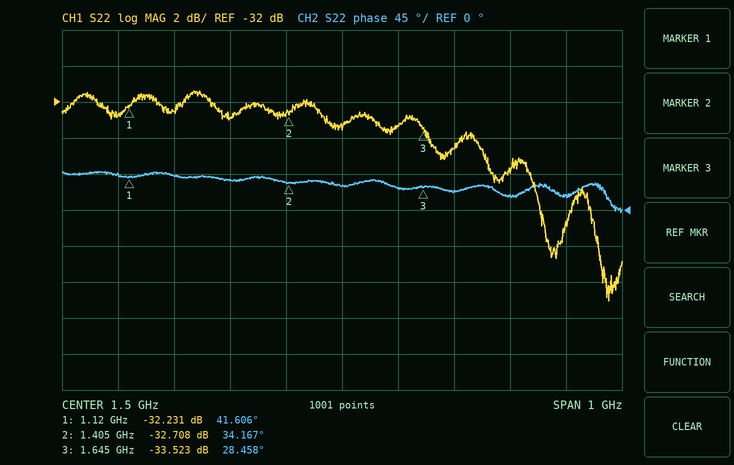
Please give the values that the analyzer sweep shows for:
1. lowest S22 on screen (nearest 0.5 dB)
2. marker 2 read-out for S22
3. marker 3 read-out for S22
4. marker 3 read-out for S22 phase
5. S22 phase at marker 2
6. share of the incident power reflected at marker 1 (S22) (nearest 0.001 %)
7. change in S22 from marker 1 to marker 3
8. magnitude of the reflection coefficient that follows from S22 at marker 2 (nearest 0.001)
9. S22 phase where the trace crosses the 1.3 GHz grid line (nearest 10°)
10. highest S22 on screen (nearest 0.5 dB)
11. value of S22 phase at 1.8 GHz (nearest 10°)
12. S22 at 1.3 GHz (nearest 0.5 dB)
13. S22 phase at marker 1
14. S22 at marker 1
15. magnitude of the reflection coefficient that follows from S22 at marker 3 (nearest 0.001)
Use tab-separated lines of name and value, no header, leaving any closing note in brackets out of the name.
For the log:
lowest S22 on screen	-43.0 dB
marker 2 read-out for S22	-32.708 dB
marker 3 read-out for S22	-33.523 dB
marker 3 read-out for S22 phase	28.458°
S22 phase at marker 2	34.167°
share of the incident power reflected at marker 1 (S22)	0.060 %
change in S22 from marker 1 to marker 3	-1.292 dB
magnitude of the reflection coefficient that follows from S22 at marker 2	0.023
S22 phase where the trace crosses the 1.3 GHz grid line	40°
highest S22 on screen	-31.5 dB
value of S22 phase at 1.8 GHz	20°
S22 at 1.3 GHz	-33.0 dB
S22 phase at marker 1	41.606°
S22 at marker 1	-32.231 dB
magnitude of the reflection coefficient that follows from S22 at marker 3	0.021
